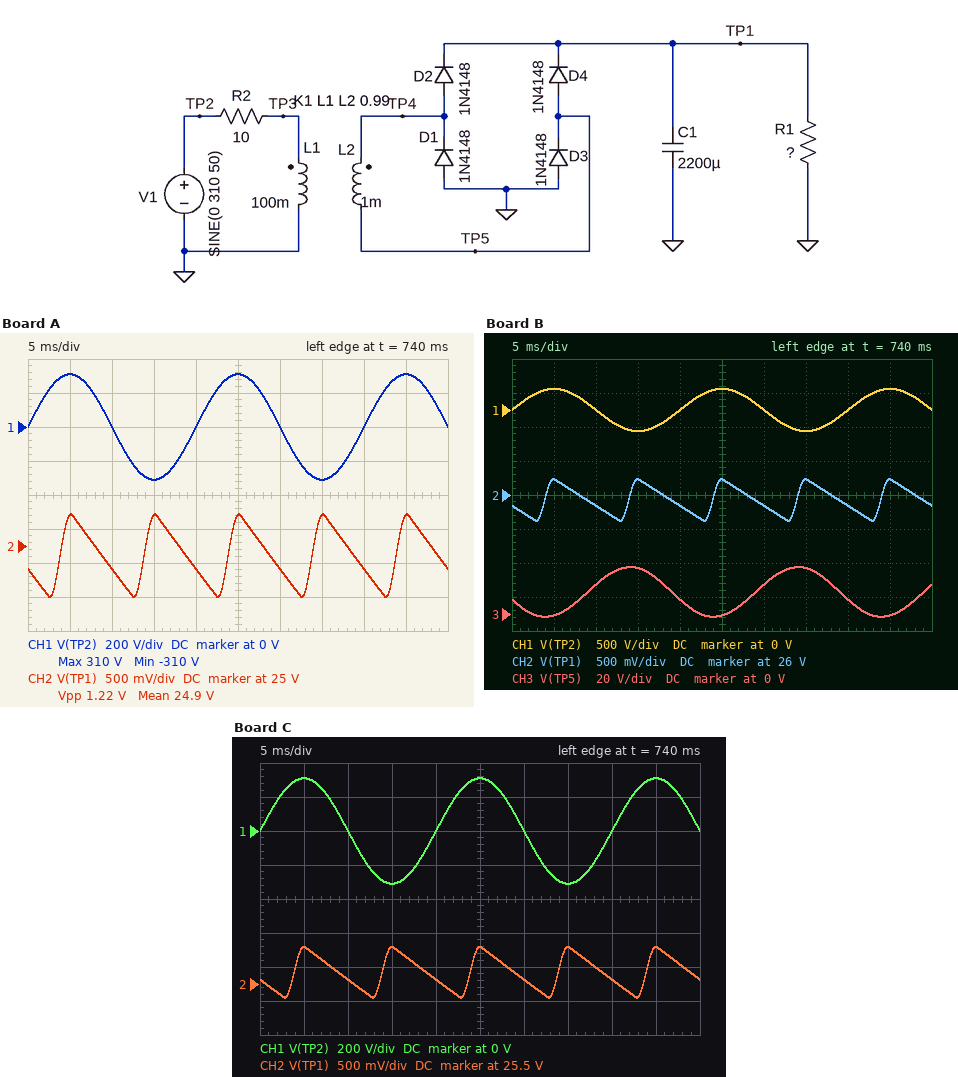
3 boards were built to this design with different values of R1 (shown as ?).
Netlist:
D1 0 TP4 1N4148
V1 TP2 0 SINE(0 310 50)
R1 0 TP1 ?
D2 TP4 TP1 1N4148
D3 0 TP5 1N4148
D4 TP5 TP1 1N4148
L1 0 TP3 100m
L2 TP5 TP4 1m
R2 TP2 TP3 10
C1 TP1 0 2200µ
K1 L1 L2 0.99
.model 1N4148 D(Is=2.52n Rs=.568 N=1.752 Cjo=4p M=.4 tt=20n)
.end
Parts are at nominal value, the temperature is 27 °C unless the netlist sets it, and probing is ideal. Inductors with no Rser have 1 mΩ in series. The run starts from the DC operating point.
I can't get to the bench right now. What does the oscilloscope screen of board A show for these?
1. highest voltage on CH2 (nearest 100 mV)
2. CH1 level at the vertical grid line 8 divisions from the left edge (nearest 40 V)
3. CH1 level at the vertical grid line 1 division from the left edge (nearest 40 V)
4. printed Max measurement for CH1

25.5 V
0 V
320 V
310 V
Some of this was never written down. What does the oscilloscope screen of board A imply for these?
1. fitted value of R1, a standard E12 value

68 Ω
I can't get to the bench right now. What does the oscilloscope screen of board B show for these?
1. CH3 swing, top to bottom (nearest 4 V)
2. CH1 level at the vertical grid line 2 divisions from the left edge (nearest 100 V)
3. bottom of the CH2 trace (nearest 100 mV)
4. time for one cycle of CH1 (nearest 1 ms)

28 V
0 V
25.6 V
20 ms
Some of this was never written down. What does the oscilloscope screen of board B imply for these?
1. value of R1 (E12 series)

150 Ω
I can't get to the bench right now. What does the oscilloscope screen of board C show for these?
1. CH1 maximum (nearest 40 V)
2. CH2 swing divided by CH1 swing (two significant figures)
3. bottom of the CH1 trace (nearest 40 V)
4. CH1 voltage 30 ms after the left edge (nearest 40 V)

320 V
0.0012
-320 V
0 V
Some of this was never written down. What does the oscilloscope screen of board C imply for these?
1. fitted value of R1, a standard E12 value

120 Ω
